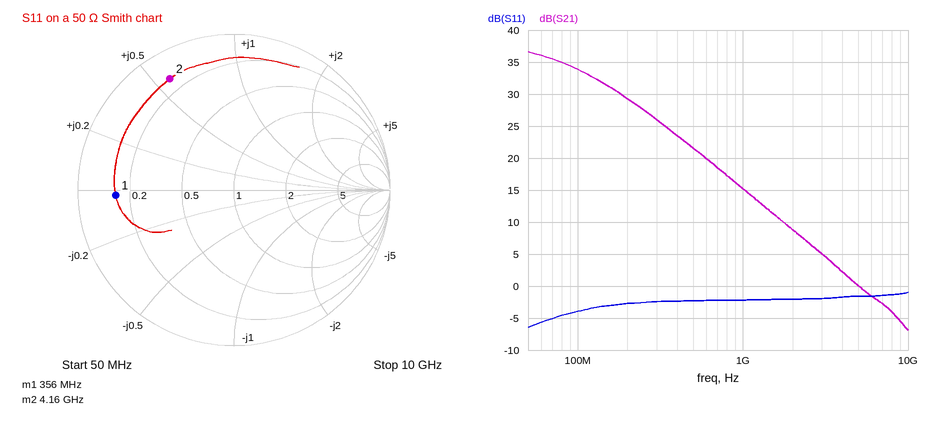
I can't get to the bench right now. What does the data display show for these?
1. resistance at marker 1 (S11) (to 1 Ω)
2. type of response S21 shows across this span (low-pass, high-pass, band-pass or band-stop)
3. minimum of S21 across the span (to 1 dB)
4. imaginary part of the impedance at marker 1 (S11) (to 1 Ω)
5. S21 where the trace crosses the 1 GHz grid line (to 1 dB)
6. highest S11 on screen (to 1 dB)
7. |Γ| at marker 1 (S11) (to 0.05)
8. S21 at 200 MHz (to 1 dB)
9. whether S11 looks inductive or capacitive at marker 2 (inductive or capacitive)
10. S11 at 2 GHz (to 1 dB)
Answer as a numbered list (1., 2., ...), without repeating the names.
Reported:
1. 7 Ω
2. low-pass
3. -7 dB
4. -1 Ω
5. 15 dB
6. -1 dB
7. 0.75
8. 29 dB
9. inductive
10. -2 dB
